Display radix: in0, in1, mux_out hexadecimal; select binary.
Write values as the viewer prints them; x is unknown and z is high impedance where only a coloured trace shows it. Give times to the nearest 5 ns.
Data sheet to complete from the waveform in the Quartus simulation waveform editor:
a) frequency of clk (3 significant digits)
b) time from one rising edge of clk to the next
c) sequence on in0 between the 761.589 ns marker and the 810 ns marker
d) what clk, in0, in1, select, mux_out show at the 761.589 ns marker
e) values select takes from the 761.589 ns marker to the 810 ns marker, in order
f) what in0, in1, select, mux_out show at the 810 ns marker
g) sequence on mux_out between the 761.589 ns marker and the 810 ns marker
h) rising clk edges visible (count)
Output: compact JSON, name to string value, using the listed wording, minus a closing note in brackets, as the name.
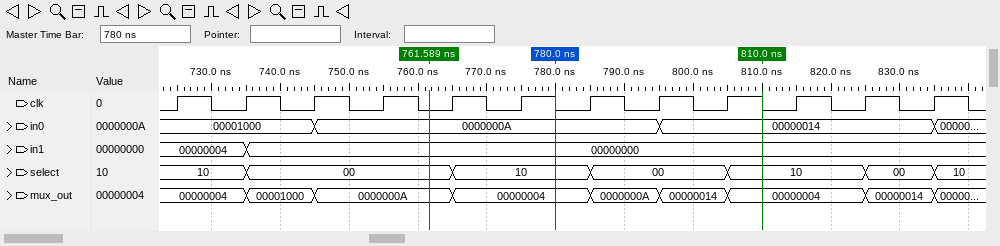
{"frequency of clk": "100 MHz", "time from one rising edge of clk to the next": "10 ns", "sequence on in0 between the 761.589 ns marker and the 810 ns marker": "0000000A, 00000014", "what clk, in0, in1, select, mux_out show at the 761.589 ns marker": "clk=0, in0=0000000A, in1=00000000, select=00, mux_out=0000000A", "values select takes from the 761.589 ns marker to the 810 ns marker, in order": "00, 10, 00, 10", "what in0, in1, select, mux_out show at the 810 ns marker": "in0=00000014, in1=00000000, select=10, mux_out=00000004", "sequence on mux_out between the 761.589 ns marker and the 810 ns marker": "0000000A, 00000004, 0000000A, 00000014, 00000004", "rising clk edges visible": "12"}
